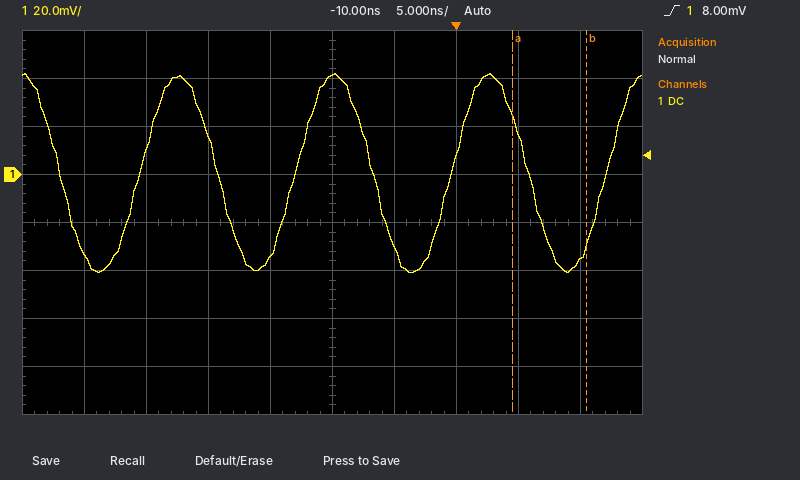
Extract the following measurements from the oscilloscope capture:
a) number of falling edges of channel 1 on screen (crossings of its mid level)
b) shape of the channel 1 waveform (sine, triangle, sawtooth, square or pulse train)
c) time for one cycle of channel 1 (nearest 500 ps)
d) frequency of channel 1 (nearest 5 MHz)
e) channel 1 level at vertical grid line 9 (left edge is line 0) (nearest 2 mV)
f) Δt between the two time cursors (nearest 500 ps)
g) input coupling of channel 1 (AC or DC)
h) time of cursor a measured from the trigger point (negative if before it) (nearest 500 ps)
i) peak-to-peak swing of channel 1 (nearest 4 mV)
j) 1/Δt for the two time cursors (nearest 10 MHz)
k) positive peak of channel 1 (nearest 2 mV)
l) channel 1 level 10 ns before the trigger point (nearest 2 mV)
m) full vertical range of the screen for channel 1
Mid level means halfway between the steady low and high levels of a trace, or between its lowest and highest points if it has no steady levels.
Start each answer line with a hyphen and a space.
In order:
- 4
- sine
- 12.5 ns
- 80 MHz
- -36 mV
- 6.0 ns
- DC
- +4.5 ns
- 84 mV
- 170 MHz
- 42 mV
- 42 mV
- 160 mV
